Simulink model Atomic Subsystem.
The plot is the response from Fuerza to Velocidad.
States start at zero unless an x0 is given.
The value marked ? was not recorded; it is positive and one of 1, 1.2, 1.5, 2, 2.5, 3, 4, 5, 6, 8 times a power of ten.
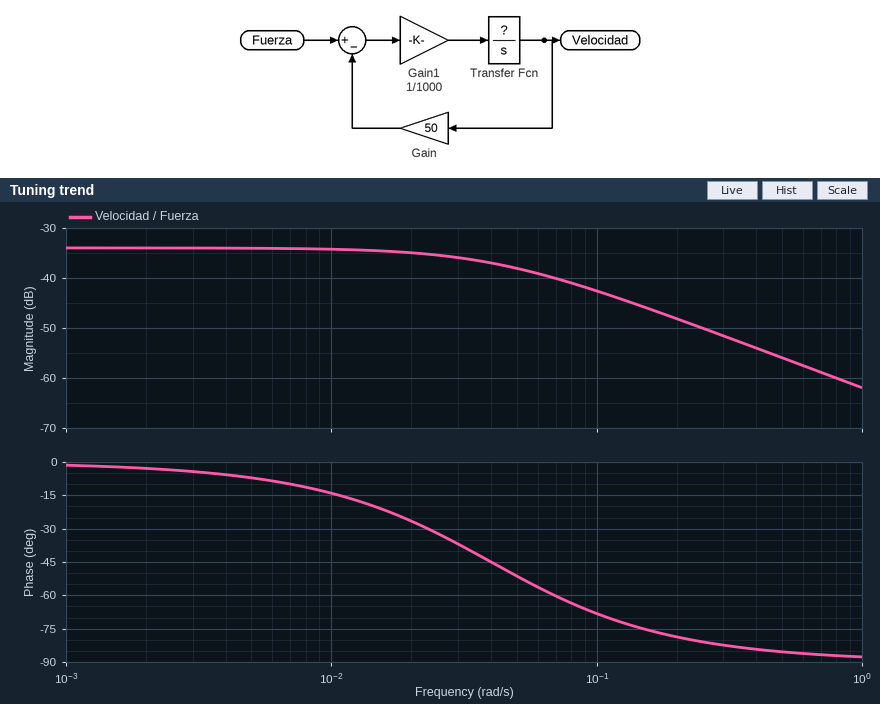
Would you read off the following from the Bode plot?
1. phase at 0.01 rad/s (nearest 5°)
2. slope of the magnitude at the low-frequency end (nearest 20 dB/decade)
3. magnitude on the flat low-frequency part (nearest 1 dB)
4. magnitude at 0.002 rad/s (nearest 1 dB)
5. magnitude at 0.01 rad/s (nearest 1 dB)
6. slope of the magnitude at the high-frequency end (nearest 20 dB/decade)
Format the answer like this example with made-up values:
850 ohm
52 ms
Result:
-15°
0 dB/decade
-34 dB
-34 dB
-34 dB
-20 dB/decade
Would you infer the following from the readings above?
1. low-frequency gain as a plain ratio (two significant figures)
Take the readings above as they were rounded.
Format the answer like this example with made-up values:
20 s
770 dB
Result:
0.020
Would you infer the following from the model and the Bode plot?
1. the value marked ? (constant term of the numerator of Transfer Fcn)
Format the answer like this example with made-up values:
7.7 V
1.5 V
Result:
0.8
